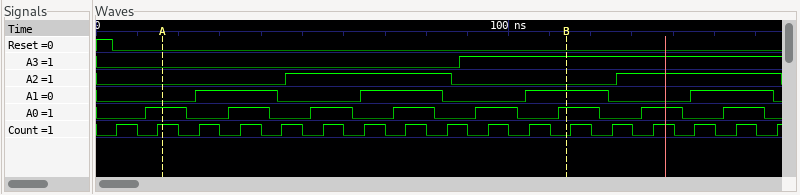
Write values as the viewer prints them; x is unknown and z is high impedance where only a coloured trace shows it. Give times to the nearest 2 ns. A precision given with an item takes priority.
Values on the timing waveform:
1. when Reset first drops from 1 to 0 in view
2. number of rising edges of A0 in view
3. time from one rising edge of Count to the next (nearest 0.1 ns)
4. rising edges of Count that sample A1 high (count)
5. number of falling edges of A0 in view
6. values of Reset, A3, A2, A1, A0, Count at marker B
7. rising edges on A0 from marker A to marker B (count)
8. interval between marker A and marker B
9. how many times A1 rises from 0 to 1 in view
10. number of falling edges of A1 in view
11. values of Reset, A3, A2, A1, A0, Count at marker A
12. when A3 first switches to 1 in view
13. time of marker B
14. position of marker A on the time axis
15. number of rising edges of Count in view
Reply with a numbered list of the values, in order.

1. 4 ns
2. 8
3. 10 ns
4. 8
5. 8
6. Reset=0, A3=1, A2=0, A1=1, A0=1, Count=0
7. 5
8. 98 ns
9. 4
10. 4
11. Reset=0, A3=0, A2=0, A1=0, A0=1, Count=1
12. 88 ns
13. 114 ns
14. 16 ns
15. 17
